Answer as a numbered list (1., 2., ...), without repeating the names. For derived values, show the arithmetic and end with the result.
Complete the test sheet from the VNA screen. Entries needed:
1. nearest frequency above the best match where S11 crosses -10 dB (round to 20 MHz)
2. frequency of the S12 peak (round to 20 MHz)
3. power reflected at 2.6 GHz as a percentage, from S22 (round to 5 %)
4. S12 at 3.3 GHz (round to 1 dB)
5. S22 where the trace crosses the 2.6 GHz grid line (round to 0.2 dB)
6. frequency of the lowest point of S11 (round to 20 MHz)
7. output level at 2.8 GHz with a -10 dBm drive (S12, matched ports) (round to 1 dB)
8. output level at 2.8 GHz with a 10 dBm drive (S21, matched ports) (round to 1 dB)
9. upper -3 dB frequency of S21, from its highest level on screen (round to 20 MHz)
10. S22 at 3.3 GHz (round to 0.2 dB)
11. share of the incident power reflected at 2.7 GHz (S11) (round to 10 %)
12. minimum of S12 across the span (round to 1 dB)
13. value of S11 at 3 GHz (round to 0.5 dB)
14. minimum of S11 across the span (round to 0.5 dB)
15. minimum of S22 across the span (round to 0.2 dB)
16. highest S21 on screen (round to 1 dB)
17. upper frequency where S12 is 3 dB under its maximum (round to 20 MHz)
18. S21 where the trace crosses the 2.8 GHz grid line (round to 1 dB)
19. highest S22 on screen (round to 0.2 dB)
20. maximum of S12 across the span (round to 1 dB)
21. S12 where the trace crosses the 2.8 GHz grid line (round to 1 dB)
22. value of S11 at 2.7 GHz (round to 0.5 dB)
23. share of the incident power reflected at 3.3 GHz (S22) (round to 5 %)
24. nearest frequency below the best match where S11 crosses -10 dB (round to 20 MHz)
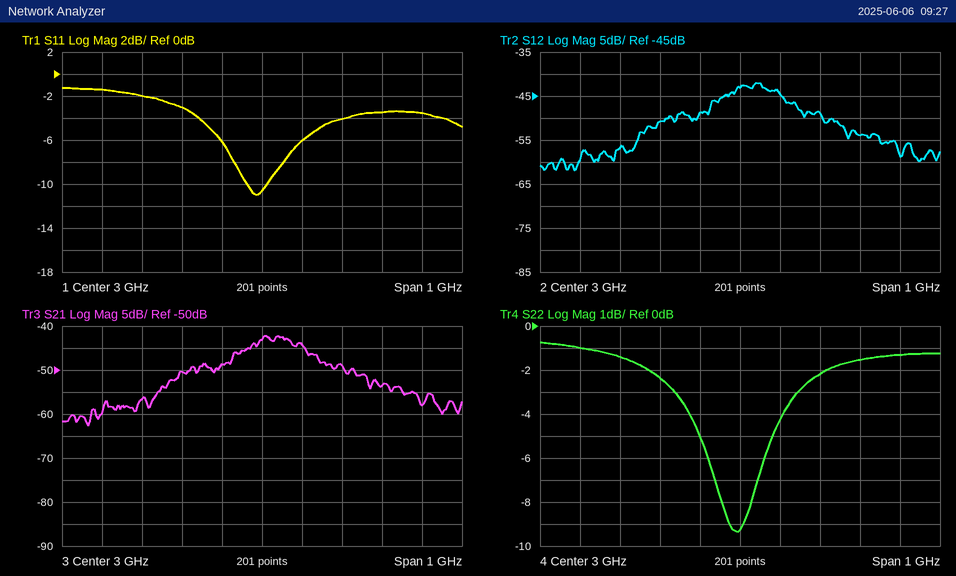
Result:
1. 3.02 GHz
2. 3.04 GHz
3. 10^(-1/10) ≈ 79.4 %, so 80 % to the nearest 5 %
4. -54 dB
5. -1.0 dB
6. 2.98 GHz
7. -10 dBm + (-51 dB) = -61 dBm
8. 10 dBm + (-50 dB) = -40 dBm
9. 3.10 GHz
10. -1.6 dB
11. 10^(-2/10) ≈ 63.1 %, so 60 % to the nearest 10 %
12. -62 dB
13. -10.5 dB
14. -11.0 dB
15. -9.4 dB
16. -42 dB
17. 3.10 GHz
18. -50 dB
19. -0.8 dB
20. -42 dB
21. -51 dB
22. -2.0 dB
23. 10^(-1.6/10) ≈ 69.2 %, so 70 % to the nearest 5 %
24. 2.96 GHz
